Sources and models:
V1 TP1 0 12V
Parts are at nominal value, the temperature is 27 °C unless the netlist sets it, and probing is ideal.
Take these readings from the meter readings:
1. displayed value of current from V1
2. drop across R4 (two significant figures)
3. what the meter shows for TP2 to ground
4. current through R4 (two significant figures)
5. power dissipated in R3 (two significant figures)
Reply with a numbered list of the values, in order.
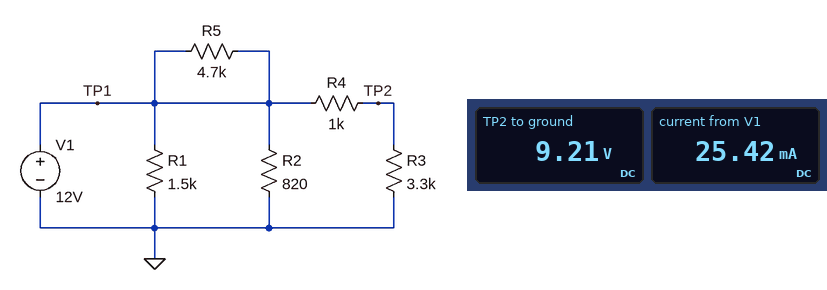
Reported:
1. 25.42 mA
2. 2.8 V
3. 9.21 V
4. 2.8 mA
5. 26 mW
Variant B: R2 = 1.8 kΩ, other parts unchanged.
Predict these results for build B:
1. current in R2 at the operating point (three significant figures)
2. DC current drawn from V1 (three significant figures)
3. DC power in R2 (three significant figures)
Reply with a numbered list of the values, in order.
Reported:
1. 6.67 mA
2. 17.5 mA
3. 80.0 mW
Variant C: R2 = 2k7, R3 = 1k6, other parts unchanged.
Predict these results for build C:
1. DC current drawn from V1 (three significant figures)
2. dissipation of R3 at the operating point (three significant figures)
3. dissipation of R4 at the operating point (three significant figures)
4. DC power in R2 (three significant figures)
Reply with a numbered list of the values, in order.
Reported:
1. 17.1 mA
2. 34.1 mW
3. 21.3 mW
4. 53.3 mW
